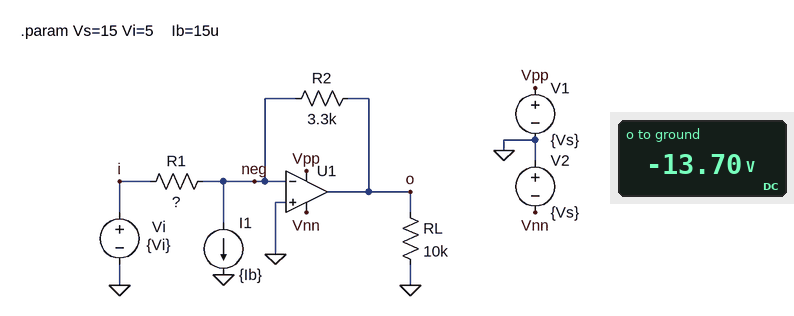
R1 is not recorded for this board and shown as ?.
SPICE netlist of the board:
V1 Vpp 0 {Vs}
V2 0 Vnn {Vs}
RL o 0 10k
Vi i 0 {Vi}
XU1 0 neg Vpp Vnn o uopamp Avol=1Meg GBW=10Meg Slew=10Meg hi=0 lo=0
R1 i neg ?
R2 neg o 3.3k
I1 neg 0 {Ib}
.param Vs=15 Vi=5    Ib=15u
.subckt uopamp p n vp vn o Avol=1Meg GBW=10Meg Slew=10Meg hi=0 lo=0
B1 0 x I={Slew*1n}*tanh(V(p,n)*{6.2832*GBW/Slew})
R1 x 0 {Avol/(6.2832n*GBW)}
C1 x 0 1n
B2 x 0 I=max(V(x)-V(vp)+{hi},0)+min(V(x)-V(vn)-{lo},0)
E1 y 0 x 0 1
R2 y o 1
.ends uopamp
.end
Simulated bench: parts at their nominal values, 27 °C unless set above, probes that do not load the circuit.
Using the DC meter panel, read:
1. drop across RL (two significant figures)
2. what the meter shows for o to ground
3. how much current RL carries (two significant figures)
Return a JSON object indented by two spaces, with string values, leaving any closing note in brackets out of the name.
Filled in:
{
  "drop across RL": "14 V",
  "what the meter shows for o to ground": "-13.70 V",
  "how much current RL carries": "1.4 mA"
}
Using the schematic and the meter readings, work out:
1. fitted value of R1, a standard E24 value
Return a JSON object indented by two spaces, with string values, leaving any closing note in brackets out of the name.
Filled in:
{
  "fitted value of R1, a standard E24 value": "1.2 kΩ"
}
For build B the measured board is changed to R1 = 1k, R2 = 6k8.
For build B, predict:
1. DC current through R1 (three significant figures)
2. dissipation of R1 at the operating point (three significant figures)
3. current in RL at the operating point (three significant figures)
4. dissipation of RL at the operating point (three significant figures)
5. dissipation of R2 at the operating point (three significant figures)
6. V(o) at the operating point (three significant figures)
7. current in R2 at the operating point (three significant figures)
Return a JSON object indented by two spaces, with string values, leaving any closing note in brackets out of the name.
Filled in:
{
  "DC current through R1": "2.58 mA",
  "dissipation of R1 at the operating point": "6.65 mW",
  "current in RL at the operating point": "1.50 mA",
  "dissipation of RL at the operating point": "22.5 mW",
  "dissipation of R2 at the operating point": "44.7 mW",
  "V(o) at the operating point": "-15.0 V",
  "current in R2 at the operating point": "2.56 mA"
}
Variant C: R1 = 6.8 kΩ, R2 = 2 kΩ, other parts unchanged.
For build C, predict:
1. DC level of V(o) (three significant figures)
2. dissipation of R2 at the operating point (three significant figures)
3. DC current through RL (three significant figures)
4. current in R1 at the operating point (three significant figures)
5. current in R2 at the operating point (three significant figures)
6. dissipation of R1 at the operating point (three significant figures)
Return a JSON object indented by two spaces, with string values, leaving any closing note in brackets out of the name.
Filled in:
{
  "DC level of V(o)": "-1.44 V",
  "dissipation of R2 at the operating point": "1.04 mW",
  "DC current through RL": "144 µA",
  "current in R1 at the operating point": "735 µA",
  "current in R2 at the operating point": "720 µA",
  "dissipation of R1 at the operating point": "3.68 mW"
}
